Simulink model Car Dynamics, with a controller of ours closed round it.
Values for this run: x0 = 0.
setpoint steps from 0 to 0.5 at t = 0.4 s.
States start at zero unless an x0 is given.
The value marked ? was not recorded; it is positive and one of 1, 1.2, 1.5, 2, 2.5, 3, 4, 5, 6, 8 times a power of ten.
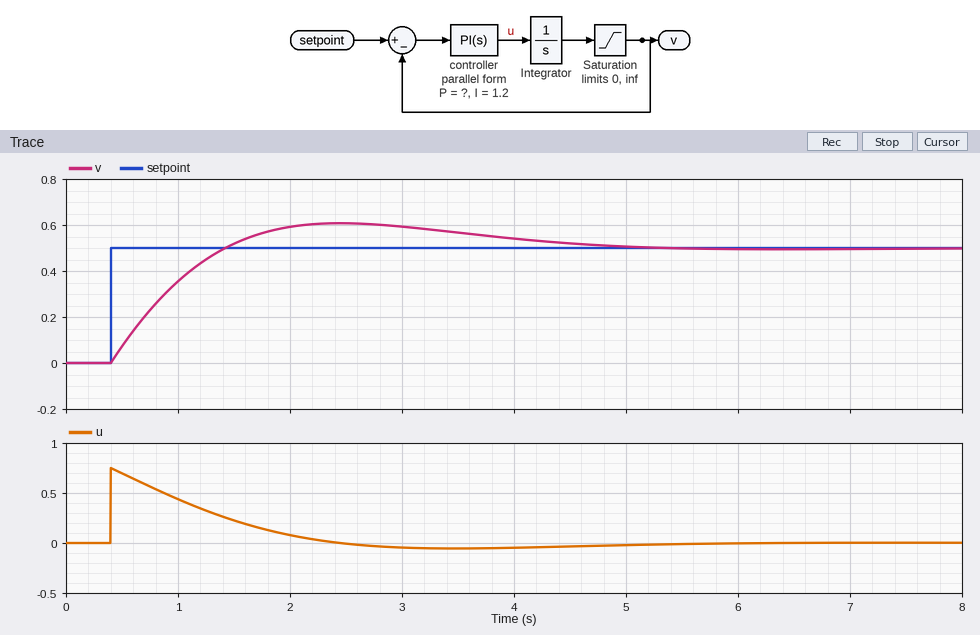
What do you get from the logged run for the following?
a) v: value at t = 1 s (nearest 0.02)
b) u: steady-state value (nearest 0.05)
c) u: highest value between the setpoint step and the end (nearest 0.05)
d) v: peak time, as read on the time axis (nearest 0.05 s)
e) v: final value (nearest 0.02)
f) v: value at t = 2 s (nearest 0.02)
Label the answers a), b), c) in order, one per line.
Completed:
a) 0.36
b) 0.00
c) 0.75
d) 2.45 s
e) 0.50
f) 0.60
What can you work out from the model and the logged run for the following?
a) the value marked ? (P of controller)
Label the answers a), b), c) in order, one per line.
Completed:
a) 1.5
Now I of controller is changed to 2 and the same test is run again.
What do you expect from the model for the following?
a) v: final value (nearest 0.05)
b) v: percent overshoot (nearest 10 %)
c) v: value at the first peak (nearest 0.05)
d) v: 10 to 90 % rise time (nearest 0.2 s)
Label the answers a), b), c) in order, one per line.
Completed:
a) 0.50
b) 30 %
c) 0.65
d) 0.6 s
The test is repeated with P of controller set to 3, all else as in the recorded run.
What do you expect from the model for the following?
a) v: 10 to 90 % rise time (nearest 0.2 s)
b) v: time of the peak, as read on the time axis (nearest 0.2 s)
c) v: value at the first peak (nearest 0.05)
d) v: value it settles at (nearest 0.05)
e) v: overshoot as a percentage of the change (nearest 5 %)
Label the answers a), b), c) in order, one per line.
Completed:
a) 0.6 s
b) 2.0 s
c) 0.55
d) 0.50
e) 10 %
